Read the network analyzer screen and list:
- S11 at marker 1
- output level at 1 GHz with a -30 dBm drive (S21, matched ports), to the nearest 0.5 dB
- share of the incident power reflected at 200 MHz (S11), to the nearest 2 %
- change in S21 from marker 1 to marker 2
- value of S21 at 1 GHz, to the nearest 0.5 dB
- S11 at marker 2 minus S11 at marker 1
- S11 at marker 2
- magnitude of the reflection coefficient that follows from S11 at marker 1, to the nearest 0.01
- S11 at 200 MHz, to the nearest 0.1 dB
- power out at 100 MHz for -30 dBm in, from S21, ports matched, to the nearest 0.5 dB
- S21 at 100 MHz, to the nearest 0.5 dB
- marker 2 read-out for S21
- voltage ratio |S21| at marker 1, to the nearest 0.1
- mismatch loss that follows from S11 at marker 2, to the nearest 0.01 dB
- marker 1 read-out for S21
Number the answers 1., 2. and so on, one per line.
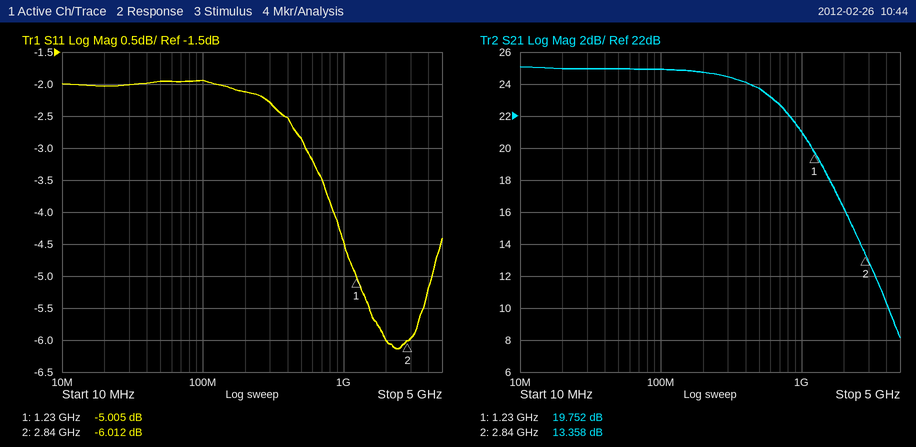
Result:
1. -5.005 dB
2. -9.0 dBm
3. 62 %
4. -6.394 dB
5. 21.0 dB
6. -1.007 dB
7. -6.012 dB
8. 0.56
9. -2.1 dB
10. -5.0 dBm
11. 25.0 dB
12. 13.358 dB
13. 9.7
14. 1.25 dB
15. 19.752 dB
